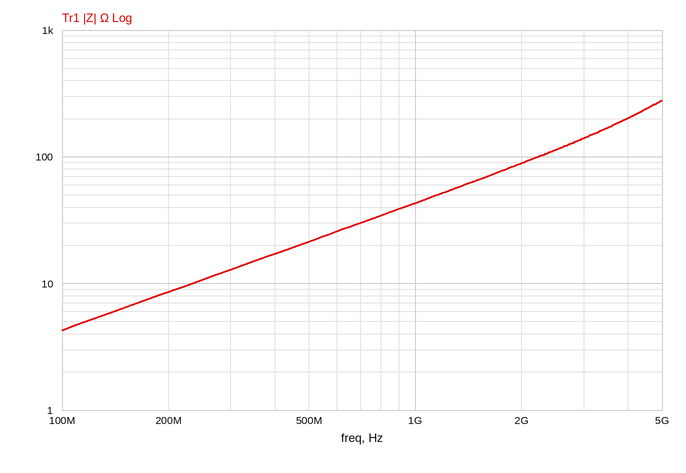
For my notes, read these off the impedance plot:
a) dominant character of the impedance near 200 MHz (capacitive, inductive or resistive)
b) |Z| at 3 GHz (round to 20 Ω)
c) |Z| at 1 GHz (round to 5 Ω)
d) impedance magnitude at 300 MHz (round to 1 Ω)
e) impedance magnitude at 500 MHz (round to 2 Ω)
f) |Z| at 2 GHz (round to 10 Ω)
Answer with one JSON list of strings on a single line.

["inductive", "140 Ω", "45 Ω", "13 Ω", "22 Ω", "90 Ω"]
